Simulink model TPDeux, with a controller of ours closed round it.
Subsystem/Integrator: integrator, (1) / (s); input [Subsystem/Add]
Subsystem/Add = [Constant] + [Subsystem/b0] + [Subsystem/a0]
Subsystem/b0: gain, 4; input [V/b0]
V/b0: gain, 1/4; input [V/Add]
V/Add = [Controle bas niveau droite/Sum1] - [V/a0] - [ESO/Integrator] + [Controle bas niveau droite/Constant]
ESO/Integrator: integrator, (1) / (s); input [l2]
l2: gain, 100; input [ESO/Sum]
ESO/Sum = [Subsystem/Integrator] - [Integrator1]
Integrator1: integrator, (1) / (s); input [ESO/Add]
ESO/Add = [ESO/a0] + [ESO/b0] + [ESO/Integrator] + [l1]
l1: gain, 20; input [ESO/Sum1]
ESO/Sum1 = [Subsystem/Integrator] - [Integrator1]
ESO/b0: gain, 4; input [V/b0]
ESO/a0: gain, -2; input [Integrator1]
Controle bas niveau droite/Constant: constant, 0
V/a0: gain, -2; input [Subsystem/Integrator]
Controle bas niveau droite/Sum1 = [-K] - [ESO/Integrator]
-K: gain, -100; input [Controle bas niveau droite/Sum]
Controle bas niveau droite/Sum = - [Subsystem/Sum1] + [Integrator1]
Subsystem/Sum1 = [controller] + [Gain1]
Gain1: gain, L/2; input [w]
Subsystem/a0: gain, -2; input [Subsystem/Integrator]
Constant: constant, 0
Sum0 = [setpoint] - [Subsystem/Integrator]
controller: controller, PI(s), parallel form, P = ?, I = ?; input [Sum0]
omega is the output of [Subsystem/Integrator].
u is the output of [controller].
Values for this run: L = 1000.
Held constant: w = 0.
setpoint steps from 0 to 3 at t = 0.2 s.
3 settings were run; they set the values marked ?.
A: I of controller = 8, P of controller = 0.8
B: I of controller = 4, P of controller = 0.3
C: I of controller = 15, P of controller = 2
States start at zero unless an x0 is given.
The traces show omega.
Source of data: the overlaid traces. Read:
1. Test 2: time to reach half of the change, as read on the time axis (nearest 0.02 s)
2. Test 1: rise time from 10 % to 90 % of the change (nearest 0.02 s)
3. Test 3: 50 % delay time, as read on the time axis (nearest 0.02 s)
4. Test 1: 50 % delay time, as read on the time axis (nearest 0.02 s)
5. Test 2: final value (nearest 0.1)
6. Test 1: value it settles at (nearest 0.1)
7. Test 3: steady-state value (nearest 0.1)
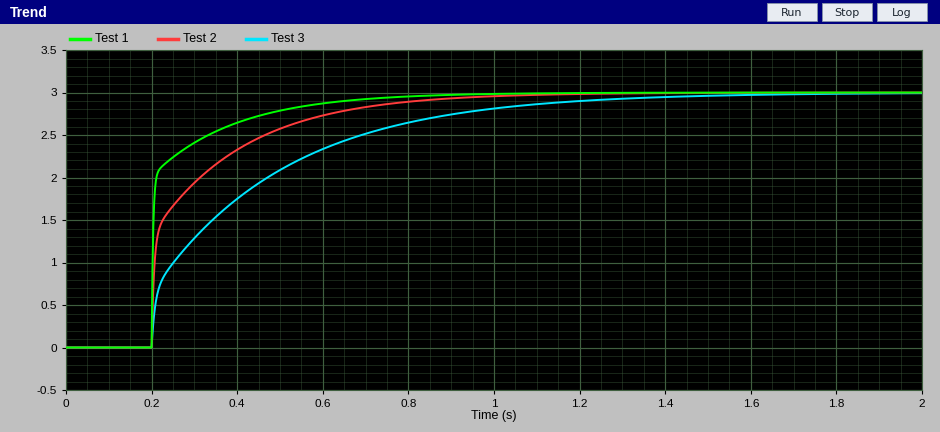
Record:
0.22 s
0.24 s
0.34 s
0.20 s
3.0
3.0
3.0
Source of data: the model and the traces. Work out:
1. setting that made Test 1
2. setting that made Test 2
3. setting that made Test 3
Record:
C
A
B
